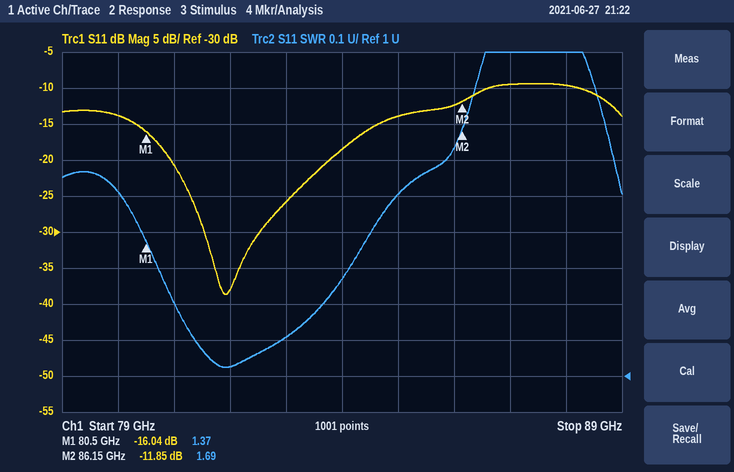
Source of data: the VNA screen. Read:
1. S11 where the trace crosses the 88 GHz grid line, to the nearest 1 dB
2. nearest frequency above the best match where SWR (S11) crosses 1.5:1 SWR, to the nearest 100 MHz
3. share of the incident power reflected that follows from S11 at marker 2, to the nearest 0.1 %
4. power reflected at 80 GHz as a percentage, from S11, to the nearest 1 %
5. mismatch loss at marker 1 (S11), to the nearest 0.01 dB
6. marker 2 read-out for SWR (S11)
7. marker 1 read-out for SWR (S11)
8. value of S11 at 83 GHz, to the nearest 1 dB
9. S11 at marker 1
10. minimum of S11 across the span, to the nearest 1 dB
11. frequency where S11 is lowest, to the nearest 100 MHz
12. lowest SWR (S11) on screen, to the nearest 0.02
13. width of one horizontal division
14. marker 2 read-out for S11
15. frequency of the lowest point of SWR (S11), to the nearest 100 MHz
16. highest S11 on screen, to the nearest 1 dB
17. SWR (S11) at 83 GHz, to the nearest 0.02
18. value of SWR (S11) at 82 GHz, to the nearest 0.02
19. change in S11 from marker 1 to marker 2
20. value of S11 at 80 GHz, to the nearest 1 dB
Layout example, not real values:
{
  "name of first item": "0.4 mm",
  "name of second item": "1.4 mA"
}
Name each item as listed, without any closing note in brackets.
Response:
{
  "S11 where the trace crosses the 88 GHz grid line, to the nearest 1 dB": "-10 dB",
  "nearest frequency above the best match where SWR (S11) crosses 1.5:1 SWR, to the nearest 100 MHz": "85.0 GHz",
  "share of the incident power reflected that follows from S11 at marker 2, to the nearest 0.1 %": "6.5 %",
  "power reflected at 80 GHz as a percentage, from S11, to the nearest 1 %": "4 %",
  "mismatch loss at marker 1 (S11), to the nearest 0.01 dB": "0.11 dB",
  "marker 2 read-out for SWR": "1.69",
  "marker 1 read-out for SWR": "1.37",
  "value of S11 at 83 GHz, to the nearest 1 dB": "-26 dB",
  "S11 at marker 1": "-16.04 dB",
  "minimum of S11 across the span, to the nearest 1 dB": "-39 dB",
  "frequency where S11 is lowest, to the nearest 100 MHz": "81.9 GHz",
  "lowest SWR (S11) on screen, to the nearest 0.02": "1.02",
  "width of one horizontal division": "1 GHz",
  "marker 2 read-out for S11": "-11.85 dB",
  "frequency of the lowest point of SWR (S11), to the nearest 100 MHz": "81.9 GHz",
  "highest S11 on screen, to the nearest 1 dB": "-9 dB",
  "SWR (S11) at 83 GHz, to the nearest 0.02": "1.10",
  "value of SWR (S11) at 82 GHz, to the nearest 0.02": "1.02",
  "change in S11 from marker 1 to marker 2": "4.19 dB",
  "value of S11 at 80 GHz, to the nearest 1 dB": "-14 dB"
}
